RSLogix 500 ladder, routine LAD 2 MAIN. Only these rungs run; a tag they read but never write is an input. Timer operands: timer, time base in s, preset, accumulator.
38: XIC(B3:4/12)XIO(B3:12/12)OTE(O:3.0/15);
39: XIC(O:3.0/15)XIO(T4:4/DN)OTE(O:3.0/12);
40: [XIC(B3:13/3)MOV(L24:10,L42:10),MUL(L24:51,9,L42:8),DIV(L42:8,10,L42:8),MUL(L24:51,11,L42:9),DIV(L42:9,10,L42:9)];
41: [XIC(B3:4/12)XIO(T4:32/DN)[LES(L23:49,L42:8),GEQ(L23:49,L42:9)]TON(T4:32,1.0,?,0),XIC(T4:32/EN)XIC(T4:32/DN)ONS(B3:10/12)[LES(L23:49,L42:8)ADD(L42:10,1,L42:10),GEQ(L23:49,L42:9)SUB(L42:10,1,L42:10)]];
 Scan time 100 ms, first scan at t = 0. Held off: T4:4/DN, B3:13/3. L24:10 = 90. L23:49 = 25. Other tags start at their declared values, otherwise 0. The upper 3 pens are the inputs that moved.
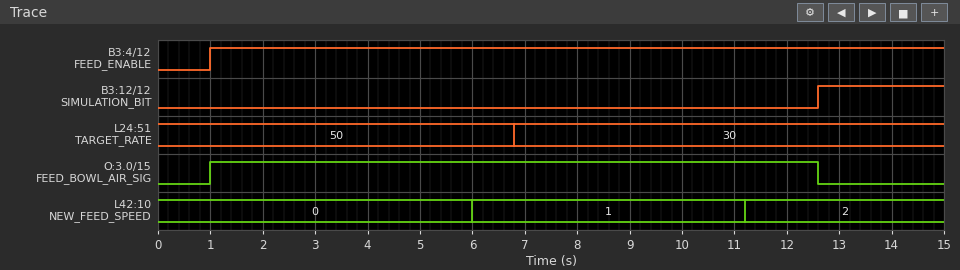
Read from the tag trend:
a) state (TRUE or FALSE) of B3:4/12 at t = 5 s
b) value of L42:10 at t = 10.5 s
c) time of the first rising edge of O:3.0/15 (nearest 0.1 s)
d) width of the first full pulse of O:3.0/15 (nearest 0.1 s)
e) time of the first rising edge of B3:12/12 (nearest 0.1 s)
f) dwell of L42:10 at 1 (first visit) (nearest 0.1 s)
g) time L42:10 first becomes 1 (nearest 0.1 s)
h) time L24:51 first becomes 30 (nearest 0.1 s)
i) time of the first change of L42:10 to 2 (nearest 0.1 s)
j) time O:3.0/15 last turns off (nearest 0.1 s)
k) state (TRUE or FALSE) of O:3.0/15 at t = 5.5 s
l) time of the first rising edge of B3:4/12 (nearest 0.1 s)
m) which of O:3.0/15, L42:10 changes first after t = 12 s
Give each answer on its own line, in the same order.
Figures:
TRUE
1
1.0 s
11.6 s
12.6 s
5.2 s
6.0 s
6.8 s
11.2 s
12.6 s
TRUE
1.0 s
O:3.0/15
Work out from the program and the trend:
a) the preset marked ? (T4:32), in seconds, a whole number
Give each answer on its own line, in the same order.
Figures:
5 s
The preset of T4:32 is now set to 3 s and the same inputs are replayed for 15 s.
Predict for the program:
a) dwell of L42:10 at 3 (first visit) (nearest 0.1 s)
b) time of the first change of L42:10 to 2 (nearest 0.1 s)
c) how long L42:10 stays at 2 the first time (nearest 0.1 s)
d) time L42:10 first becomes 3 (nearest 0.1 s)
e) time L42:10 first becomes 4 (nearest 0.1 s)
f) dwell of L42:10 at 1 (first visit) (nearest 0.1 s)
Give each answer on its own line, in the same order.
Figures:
3.2 s
7.2 s
3.2 s
10.4 s
13.6 s
3.2 s
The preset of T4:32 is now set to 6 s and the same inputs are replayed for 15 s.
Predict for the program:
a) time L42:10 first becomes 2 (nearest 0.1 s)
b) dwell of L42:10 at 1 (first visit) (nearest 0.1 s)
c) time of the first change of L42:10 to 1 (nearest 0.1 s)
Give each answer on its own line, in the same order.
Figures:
13.2 s
6.2 s
7.0 s
